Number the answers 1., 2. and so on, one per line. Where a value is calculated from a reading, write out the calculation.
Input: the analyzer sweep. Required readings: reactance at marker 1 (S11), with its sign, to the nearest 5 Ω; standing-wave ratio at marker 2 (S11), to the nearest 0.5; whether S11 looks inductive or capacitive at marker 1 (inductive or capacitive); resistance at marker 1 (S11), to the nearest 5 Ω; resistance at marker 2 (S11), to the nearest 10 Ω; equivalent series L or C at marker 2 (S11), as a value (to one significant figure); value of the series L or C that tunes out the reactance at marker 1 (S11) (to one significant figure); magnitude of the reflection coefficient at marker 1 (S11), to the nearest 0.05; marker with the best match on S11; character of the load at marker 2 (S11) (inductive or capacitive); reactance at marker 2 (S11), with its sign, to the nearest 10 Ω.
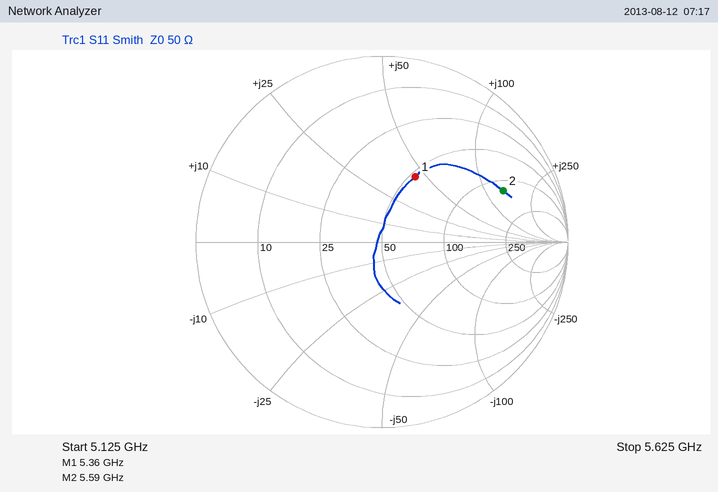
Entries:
1. +45 Ω
2. 6.0
3. inductive
4. 55 Ω
5. 130 Ω
6. L = 140 Ω/(2π × 5.59 GHz) ≈ 4 nH
7. C = 1/(2π × 5.36 GHz × 45 Ω) ≈ 660 fF, so 700 fF to one significant figure
8. 0.40
9. marker 1
10. inductive
11. +140 Ω
